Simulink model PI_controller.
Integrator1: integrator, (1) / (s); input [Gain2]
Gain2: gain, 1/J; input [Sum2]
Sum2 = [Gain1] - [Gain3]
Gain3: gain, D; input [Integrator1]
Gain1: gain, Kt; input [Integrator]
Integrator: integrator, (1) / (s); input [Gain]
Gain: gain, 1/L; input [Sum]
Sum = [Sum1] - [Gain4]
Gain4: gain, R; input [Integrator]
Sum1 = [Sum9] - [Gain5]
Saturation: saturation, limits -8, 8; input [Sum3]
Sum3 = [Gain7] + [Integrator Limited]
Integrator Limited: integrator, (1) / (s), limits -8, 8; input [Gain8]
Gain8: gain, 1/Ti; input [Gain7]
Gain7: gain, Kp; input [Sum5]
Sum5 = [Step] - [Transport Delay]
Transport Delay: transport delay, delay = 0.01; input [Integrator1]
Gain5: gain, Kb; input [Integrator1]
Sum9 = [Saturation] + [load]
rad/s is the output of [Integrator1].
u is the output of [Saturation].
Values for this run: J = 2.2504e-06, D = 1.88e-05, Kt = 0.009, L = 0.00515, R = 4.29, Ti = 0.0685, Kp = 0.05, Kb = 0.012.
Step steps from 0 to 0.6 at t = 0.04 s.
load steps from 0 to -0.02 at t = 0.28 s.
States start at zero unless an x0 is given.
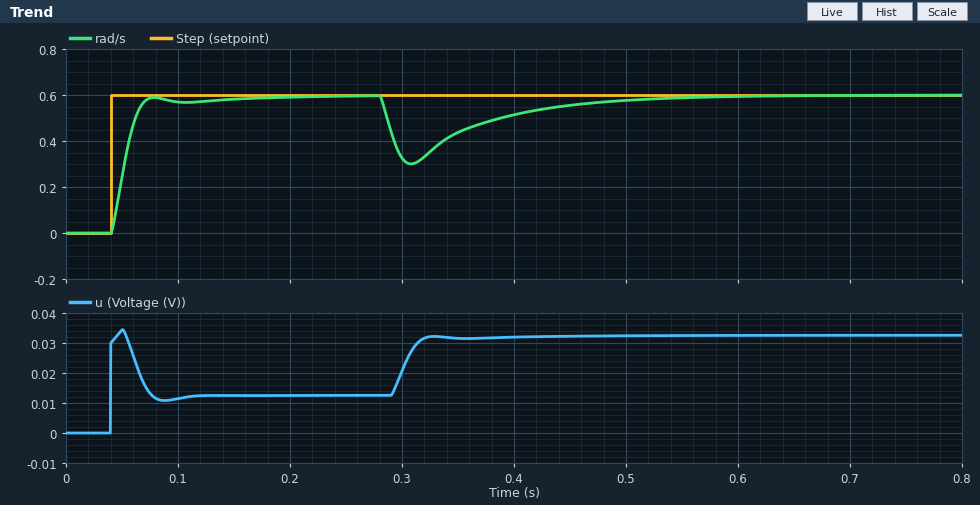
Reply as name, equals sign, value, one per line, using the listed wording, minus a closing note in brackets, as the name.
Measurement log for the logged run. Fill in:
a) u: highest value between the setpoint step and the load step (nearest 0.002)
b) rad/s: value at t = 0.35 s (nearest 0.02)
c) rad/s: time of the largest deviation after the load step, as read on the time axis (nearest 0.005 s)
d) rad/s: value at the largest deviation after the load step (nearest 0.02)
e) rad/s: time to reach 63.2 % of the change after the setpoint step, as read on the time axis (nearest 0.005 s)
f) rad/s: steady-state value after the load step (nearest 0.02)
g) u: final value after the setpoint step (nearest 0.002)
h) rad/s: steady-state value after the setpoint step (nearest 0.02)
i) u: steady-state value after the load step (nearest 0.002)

u: highest value between the setpoint step and the load step = 0.034
rad/s: value at t = 0.35 s = 0.44
rad/s: time of the largest deviation after the load step, as read on the time axis = 0.310 s
rad/s: value at the largest deviation after the load step = 0.30
rad/s: time to reach 63.2 % of the change after the setpoint step, as read on the time axis = 0.055 s
rad/s: steady-state value after the load step = 0.60
u: final value after the setpoint step = 0.012
rad/s: steady-state value after the setpoint step = 0.60
u: steady-state value after the load step = 0.032
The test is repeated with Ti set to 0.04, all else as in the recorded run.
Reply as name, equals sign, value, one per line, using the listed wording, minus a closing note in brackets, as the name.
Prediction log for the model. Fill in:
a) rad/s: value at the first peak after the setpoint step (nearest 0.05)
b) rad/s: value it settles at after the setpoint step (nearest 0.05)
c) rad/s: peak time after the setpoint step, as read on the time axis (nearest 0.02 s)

rad/s: value at the first peak after the setpoint step = 0.70
rad/s: value it settles at after the setpoint step = 0.60
rad/s: peak time after the setpoint step, as read on the time axis = 0.08 s
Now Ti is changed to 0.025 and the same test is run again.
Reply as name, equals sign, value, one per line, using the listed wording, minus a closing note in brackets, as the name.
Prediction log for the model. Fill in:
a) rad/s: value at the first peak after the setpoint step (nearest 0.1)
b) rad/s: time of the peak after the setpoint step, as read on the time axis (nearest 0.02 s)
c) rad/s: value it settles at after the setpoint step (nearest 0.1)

rad/s: value at the first peak after the setpoint step = 0.8
rad/s: time of the peak after the setpoint step, as read on the time axis = 0.08 s
rad/s: value it settles at after the setpoint step = 0.6
